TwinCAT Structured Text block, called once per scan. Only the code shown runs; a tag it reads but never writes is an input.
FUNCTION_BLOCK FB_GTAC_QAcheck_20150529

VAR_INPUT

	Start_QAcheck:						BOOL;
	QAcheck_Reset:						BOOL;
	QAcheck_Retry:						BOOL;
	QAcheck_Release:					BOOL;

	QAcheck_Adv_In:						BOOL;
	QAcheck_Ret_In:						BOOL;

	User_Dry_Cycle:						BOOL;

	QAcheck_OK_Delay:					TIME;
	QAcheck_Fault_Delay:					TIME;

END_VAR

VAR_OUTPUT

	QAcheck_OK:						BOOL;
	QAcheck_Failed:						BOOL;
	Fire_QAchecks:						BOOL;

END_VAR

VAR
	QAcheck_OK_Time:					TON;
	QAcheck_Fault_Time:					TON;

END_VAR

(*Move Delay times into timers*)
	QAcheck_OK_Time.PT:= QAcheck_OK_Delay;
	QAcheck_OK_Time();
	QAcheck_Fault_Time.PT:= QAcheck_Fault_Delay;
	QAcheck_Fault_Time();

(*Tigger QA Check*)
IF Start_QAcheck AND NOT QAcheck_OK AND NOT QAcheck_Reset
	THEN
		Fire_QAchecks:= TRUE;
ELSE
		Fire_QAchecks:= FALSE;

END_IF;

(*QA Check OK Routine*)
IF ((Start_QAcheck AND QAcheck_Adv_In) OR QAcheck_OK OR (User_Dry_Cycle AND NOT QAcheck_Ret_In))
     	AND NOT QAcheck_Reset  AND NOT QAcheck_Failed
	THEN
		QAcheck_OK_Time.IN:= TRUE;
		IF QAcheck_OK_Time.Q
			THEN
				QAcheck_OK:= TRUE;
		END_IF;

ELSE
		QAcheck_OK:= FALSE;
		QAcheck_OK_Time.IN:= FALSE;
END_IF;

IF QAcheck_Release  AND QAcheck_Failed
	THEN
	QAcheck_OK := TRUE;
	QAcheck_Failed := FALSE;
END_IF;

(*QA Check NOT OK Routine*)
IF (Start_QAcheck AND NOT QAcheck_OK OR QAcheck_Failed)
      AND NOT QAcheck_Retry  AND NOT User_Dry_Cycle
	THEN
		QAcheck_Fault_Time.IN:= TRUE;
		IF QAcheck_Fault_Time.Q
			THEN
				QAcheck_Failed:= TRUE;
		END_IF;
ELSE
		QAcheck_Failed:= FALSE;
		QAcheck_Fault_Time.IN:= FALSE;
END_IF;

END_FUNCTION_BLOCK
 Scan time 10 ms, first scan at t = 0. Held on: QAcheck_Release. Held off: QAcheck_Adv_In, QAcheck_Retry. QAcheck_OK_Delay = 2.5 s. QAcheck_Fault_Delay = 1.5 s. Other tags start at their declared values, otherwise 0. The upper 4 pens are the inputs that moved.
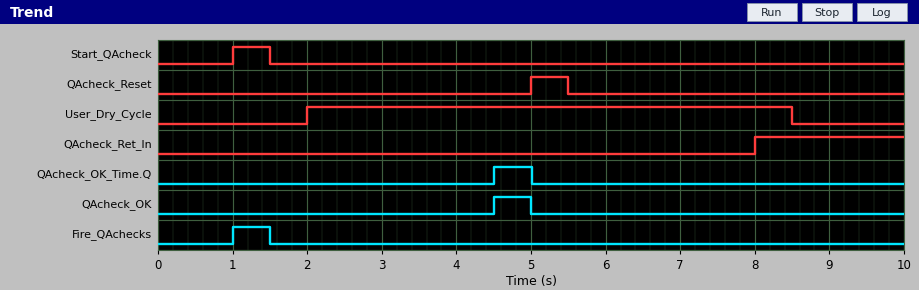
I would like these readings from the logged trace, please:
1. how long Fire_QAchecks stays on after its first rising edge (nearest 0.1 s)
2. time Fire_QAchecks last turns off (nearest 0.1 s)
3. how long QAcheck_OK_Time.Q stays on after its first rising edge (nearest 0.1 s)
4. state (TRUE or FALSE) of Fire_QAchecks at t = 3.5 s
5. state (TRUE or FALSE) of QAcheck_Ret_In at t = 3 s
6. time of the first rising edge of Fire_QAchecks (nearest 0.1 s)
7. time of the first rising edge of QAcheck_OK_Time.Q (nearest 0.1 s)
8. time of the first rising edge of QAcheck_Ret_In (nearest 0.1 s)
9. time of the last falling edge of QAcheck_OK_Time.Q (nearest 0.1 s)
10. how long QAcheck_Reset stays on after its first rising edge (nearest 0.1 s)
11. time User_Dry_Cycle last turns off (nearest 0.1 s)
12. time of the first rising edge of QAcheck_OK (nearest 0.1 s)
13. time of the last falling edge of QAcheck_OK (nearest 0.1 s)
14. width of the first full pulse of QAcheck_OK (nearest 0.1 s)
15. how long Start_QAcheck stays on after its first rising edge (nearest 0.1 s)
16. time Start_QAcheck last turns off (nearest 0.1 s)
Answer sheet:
0.5 s
1.5 s
0.5 s
FALSE
FALSE
1.0 s
4.5 s
8.0 s
5.0 s
0.5 s
8.5 s
4.5 s
5.0 s
0.5 s
0.5 s
1.5 s
